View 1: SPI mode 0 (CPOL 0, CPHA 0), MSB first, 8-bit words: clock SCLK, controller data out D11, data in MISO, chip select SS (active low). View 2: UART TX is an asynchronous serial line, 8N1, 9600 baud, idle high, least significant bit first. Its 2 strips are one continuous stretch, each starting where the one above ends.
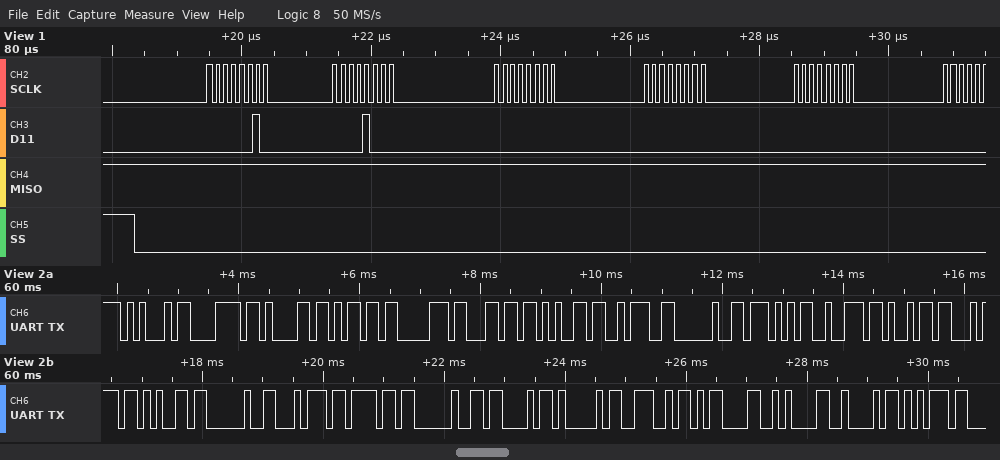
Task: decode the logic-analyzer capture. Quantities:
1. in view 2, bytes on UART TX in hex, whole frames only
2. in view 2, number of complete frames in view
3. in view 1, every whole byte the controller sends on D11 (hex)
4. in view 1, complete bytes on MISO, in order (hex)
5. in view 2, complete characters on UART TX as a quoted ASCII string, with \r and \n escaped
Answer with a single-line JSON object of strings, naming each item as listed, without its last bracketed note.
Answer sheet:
{"in view 2, bytes on UART TX in hex, whole frames only": "45 78 61 6D 70 6C 65 3A 20 57 72 69 74 65 20 74 6F 20 43 41 4E 0D 0A 42 75", "in view 2, number of complete frames in view": "25", "in view 1, every whole byte the controller sends on D11": "02 08 00 00 00", "in view 1, complete bytes on MISO, in order": "FF FF FF FF FF", "in view 2, complete characters on UART TX as a quoted ASCII string, with \\r and \\n escaped": "\"Example: Write to CAN\\r\\nBu\""}
